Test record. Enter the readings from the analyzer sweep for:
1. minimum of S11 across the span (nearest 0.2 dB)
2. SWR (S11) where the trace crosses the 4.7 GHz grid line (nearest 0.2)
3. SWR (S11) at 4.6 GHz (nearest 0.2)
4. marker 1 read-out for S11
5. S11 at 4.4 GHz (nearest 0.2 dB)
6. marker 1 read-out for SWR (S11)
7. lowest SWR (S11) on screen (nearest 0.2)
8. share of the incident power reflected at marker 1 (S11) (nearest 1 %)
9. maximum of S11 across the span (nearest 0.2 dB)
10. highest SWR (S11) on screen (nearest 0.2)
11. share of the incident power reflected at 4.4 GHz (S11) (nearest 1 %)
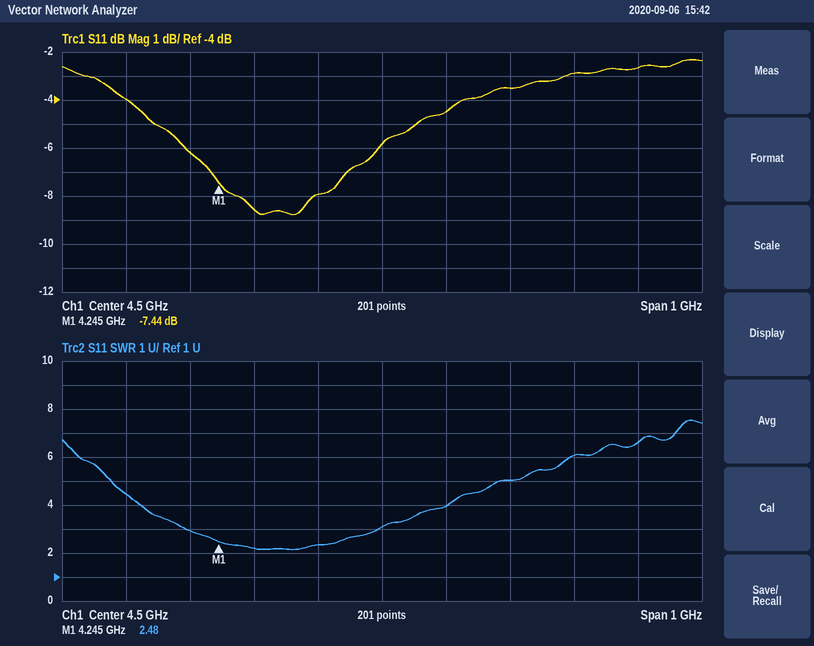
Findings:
-8.8 dB
5.0
4.0
-7.44 dB
-8.0 dB
2.48
2.2
18 %
-2.4 dB
7.6
16 %
